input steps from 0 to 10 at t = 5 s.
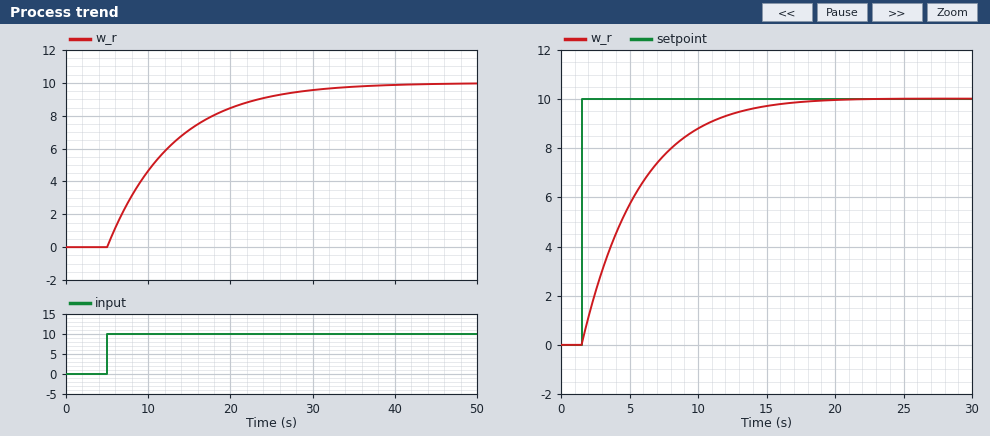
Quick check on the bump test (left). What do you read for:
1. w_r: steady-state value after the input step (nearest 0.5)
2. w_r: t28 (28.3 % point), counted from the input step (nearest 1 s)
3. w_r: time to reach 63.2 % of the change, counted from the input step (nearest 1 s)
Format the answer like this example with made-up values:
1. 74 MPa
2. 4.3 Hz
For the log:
1. 10.0
2. 3 s
3. 8 s
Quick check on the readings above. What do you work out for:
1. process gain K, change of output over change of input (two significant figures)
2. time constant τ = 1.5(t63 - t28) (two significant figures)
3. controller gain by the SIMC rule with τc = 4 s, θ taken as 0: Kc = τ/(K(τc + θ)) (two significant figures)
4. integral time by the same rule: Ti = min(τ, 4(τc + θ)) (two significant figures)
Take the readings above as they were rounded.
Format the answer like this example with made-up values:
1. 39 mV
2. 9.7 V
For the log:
1. 1.0
2. 7.5 s
3. 1.9
4. 7.5 s
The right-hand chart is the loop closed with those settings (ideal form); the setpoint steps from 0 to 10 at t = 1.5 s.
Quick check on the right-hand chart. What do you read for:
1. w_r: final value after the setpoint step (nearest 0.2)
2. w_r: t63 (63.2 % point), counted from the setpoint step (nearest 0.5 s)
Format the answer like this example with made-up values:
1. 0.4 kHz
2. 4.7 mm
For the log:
1. 10.0
2. 4.0 s
